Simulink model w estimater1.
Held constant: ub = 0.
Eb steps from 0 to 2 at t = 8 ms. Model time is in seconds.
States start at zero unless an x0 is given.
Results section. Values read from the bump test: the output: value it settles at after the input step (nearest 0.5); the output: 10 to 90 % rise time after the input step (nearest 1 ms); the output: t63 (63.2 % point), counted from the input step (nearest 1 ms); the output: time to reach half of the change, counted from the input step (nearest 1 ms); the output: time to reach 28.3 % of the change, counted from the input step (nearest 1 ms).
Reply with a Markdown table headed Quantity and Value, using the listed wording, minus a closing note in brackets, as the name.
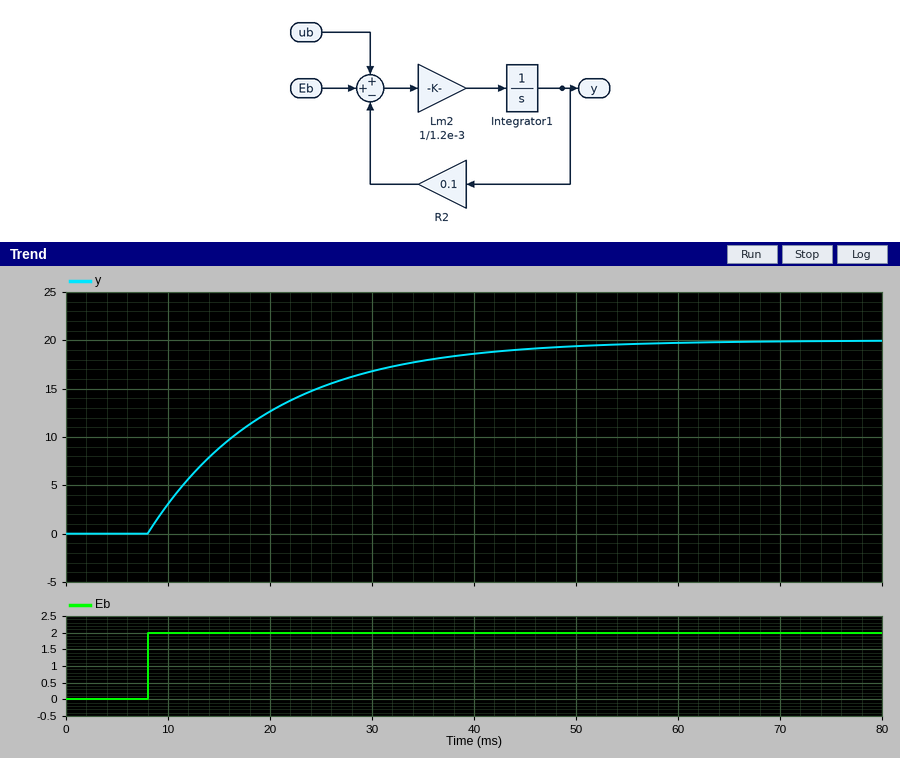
| Quantity | Value |
|---|---|
| the output: value it settles at after the input step | 20.0 |
| the output: 10 to 90 % rise time after the input step | 26 ms |
| the output: t63 (63.2 % point), counted from the input step | 12 ms |
| the output: time to reach half of the change, counted from the input step | 8 ms |
| the output: time to reach 28.3 % of the change, counted from the input step | 4 ms |
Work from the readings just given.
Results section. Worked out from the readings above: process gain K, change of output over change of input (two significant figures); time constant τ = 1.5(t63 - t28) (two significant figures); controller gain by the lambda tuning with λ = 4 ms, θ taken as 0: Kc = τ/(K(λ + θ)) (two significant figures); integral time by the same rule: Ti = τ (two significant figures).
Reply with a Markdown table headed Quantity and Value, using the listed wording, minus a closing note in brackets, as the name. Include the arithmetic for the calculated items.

| Quantity | Value |
|---|---|
| process gain K, change of output over change of input | (20 - 0) / 2 = 10 |
| time constant τ = 1.5(t63 - t28) | 1.5 × (12 - 4) = 12 ms |
| controller gain by the lambda tuning with λ = 4 ms, θ taken as 0: Kc = τ/(K(λ + θ)) | 12 / (10 × (4 + 0)) = 0.30 |
| integral time by the same rule: Ti = τ | 12 ms |
